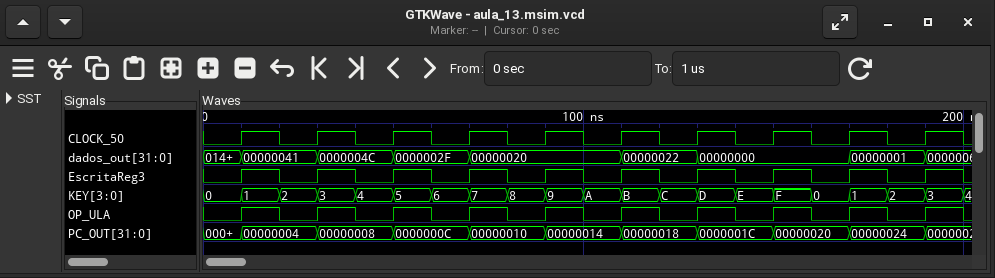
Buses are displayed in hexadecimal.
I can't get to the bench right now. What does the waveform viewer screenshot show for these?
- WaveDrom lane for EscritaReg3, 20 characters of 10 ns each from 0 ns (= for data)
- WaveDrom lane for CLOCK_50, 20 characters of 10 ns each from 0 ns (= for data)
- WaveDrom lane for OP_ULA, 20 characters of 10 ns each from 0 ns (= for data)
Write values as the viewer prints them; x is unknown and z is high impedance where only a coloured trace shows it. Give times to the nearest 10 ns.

{name: 'EscritaReg3', wave: '01010101010101010101'}
{name: 'CLOCK_50', wave: '01010101010101010101'}
{name: 'OP_ULA', wave: '01010101010101010101'}
